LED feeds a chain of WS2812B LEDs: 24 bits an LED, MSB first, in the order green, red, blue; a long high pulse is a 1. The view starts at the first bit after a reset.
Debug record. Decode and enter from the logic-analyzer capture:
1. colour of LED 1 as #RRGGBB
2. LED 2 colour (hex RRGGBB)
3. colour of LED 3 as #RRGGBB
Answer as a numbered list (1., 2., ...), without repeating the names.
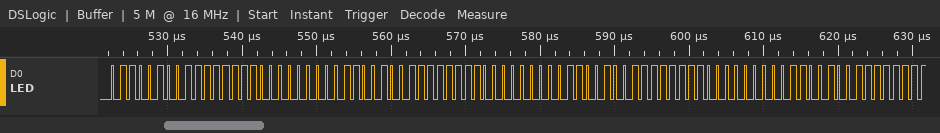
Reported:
1. #FF6400
2. #FF6400
3. #FF6400
